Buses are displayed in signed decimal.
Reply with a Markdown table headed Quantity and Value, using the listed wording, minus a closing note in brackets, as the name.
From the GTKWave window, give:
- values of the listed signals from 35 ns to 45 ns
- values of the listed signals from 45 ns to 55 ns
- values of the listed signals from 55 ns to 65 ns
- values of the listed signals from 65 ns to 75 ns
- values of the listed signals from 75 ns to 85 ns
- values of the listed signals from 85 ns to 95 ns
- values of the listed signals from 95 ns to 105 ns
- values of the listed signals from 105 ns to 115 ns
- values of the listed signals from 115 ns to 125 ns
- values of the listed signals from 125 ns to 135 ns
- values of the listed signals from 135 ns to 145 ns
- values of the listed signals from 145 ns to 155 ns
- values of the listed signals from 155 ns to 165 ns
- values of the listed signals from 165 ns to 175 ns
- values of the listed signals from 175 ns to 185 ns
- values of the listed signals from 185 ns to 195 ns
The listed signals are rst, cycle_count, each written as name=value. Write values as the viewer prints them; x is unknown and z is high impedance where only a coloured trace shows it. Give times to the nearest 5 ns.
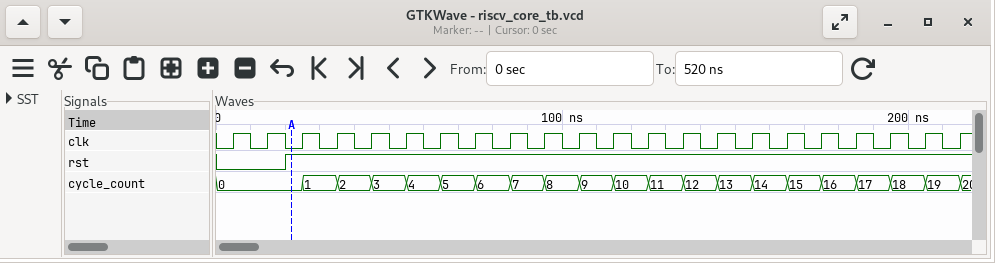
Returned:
| Quantity | Value |
|---|---|
| values of the listed signals from 35 ns to 45 ns | rst=1, cycle_count=2 |
| values of the listed signals from 45 ns to 55 ns | rst=1, cycle_count=3 |
| values of the listed signals from 55 ns to 65 ns | rst=1, cycle_count=4 |
| values of the listed signals from 65 ns to 75 ns | rst=1, cycle_count=5 |
| values of the listed signals from 75 ns to 85 ns | rst=1, cycle_count=6 |
| values of the listed signals from 85 ns to 95 ns | rst=1, cycle_count=7 |
| values of the listed signals from 95 ns to 105 ns | rst=1, cycle_count=8 |
| values of the listed signals from 105 ns to 115 ns | rst=1, cycle_count=9 |
| values of the listed signals from 115 ns to 125 ns | rst=1, cycle_count=10 |
| values of the listed signals from 125 ns to 135 ns | rst=1, cycle_count=11 |
| values of the listed signals from 135 ns to 145 ns | rst=1, cycle_count=12 |
| values of the listed signals from 145 ns to 155 ns | rst=1, cycle_count=13 |
| values of the listed signals from 155 ns to 165 ns | rst=1, cycle_count=14 |
| values of the listed signals from 165 ns to 175 ns | rst=1, cycle_count=15 |
| values of the listed signals from 175 ns to 185 ns | rst=1, cycle_count=16 |
| values of the listed signals from 185 ns to 195 ns | rst=1, cycle_count=17 |
